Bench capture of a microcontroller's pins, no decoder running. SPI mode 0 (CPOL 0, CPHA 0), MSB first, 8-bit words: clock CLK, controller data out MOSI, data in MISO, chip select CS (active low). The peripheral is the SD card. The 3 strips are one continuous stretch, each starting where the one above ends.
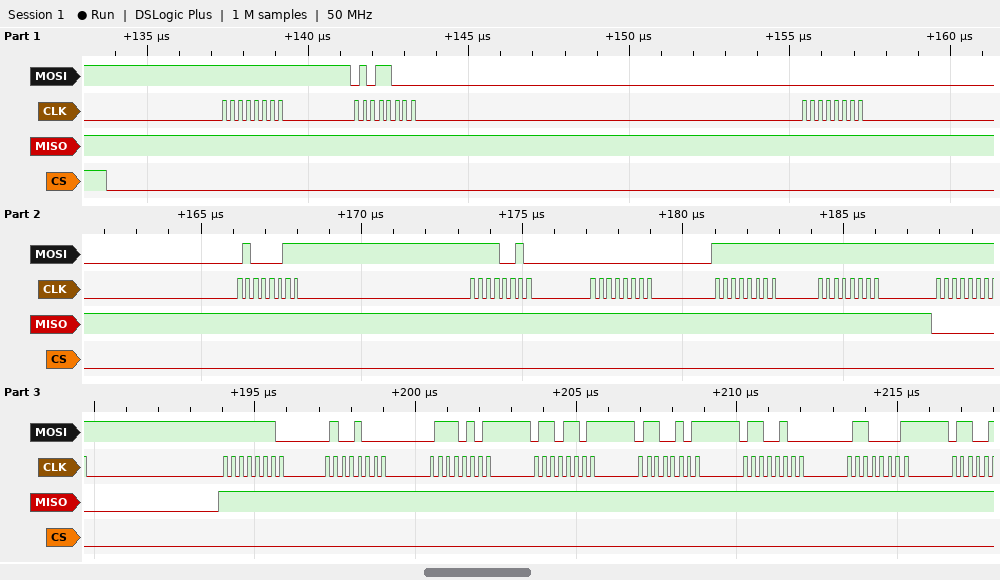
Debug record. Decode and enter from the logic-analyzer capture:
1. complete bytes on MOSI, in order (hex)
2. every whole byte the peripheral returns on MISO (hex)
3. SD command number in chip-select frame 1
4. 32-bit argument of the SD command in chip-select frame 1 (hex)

FF 58 00 43 F2 00 FF FF FF FE 48 75 6D 65 64 61
FF FF FF FF FF FF FF FF 00 FF FF FF FF FF FF FF
CMD24
0x0043F200
